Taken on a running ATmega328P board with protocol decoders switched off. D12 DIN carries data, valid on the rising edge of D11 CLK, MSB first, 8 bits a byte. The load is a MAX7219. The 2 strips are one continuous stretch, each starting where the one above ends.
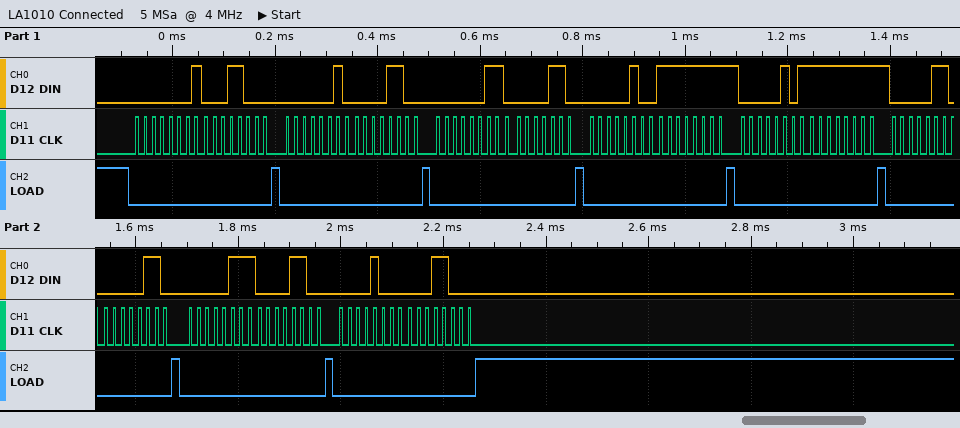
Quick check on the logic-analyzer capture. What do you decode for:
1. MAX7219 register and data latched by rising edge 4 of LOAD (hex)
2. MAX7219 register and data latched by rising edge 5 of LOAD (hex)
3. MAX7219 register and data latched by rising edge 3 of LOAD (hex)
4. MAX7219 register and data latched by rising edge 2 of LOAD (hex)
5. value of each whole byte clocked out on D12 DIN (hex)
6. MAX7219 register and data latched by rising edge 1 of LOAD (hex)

register 0x4, data 0xFF
register 0x5, data 0xFF
register 0x3, data 0x06
register 0x2, data 0x0C
01 18 02 0C 03 06 04 FF 05 FF 06 06 07 0C 08 18
register 0x1, data 0x18
